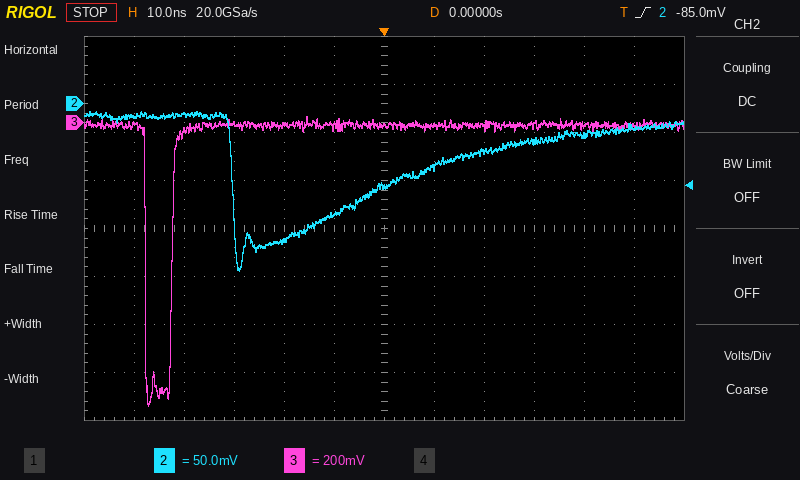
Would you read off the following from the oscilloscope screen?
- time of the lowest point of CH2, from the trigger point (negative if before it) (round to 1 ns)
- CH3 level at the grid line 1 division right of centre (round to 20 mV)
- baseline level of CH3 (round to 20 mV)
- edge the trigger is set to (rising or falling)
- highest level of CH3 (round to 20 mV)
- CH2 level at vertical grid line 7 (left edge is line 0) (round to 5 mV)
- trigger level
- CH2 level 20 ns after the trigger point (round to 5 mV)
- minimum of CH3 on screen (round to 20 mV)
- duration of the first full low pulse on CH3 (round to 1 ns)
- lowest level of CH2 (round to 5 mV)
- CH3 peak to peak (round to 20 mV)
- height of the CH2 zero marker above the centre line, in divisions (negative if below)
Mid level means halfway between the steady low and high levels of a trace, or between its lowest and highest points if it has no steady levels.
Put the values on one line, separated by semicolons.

-29 ns; -20 mV; 0 mV; rising; 20 mV; -65 mV; -85.0 mV; -50 mV; -1.18 V; 5 ns; -175 mV; 1.20 V; +2.6 div
